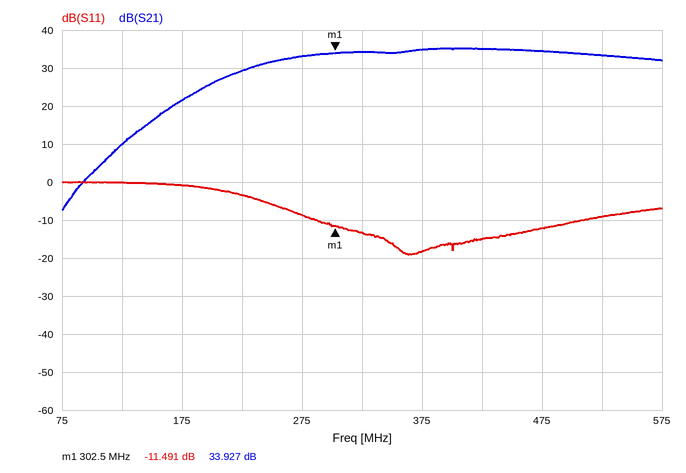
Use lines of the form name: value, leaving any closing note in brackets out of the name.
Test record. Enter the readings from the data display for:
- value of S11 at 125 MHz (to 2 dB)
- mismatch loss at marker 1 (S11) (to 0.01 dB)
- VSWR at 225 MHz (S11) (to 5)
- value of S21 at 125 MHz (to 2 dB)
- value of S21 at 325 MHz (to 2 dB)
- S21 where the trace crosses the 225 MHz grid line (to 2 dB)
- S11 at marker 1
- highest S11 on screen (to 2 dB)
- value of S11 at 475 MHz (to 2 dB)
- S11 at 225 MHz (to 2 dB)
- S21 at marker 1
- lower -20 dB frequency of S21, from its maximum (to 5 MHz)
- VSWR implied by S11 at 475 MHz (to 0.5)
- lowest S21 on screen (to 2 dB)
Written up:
value of S11 at 125 MHz: 0 dB
mismatch loss at marker 1 (S11): 0.32 dB
VSWR at 225 MHz (S11): 5
value of S21 at 125 MHz: 10 dB
value of S21 at 325 MHz: 34 dB
S21 where the trace crosses the 225 MHz grid line: 30 dB
S11 at marker 1: -11.491 dB
highest S11 on screen: 0 dB
value of S11 at 475 MHz: -12 dB
S11 at 225 MHz: -4 dB
S21 at marker 1: 33.927 dB
lower -20 dB frequency of S21, from its maximum: 145 MHz
VSWR implied by S11 at 475 MHz: 1.5
lowest S21 on screen: -8 dB
